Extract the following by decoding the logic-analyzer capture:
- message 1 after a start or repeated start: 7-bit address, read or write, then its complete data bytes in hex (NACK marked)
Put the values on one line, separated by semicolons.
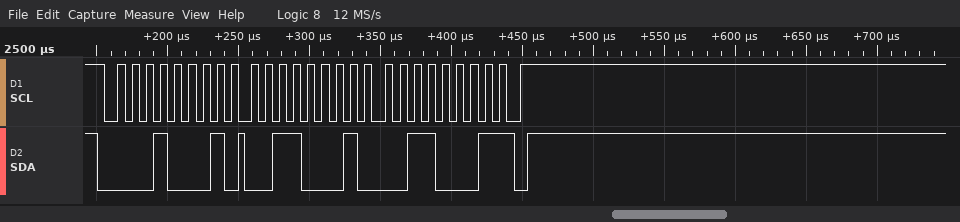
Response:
0x08 read: 31 31 NACK
